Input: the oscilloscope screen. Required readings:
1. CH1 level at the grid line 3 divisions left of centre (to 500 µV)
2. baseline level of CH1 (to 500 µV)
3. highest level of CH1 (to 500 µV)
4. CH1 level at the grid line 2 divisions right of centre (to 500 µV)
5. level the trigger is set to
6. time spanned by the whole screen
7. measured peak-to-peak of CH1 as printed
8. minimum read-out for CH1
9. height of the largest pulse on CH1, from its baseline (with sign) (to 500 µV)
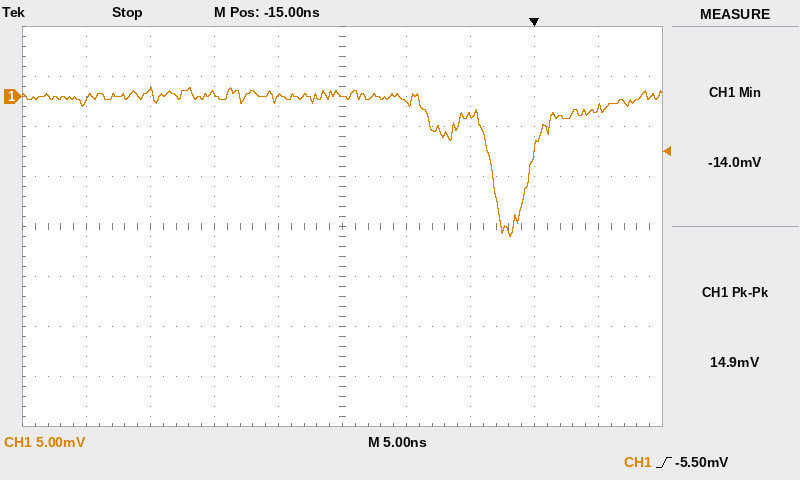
500 µV
0.0 mV
1.0 mV
-2.0 mV
-5.50 mV
50 ns
14.9 mV
-14.0 mV
-14.0 mV
